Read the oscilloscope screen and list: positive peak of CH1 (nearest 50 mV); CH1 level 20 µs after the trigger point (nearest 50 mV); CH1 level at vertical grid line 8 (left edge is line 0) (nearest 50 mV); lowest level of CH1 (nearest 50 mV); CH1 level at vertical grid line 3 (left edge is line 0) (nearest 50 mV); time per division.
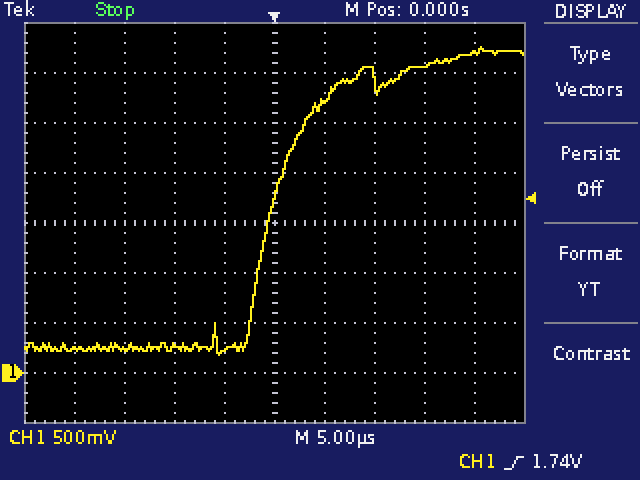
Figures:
3.25 V
3.20 V
3.05 V
200 mV
250 mV
5 µs
